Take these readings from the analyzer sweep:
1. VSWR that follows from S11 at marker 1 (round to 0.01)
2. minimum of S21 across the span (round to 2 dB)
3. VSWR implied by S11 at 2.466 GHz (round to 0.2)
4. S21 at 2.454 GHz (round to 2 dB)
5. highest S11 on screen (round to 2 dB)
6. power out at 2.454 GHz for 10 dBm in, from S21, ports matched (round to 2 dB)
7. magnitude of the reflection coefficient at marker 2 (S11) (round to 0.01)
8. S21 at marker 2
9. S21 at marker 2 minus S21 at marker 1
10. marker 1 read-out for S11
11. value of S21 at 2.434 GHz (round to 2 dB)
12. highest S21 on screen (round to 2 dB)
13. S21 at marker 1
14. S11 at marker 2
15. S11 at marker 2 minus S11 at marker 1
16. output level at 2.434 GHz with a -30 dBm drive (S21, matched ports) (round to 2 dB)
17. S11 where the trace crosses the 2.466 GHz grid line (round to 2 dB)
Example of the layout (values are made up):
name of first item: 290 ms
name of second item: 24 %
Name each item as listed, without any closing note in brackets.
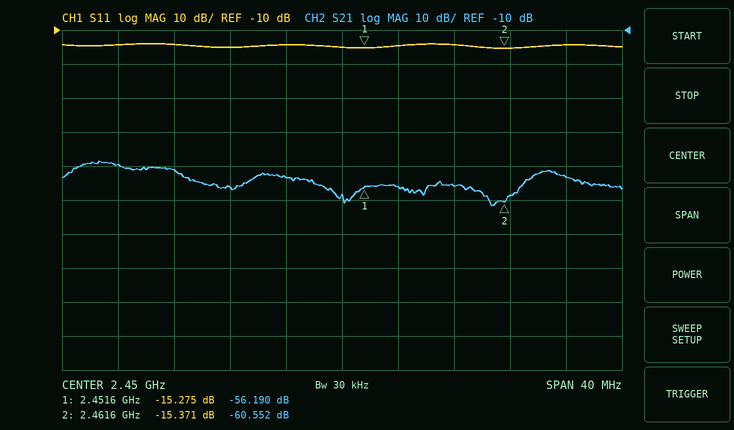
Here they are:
VSWR that follows from S11 at marker 1: 1.42
minimum of S21 across the span: -62 dB
VSWR implied by S11 at 2.466 GHz: 1.4
S21 at 2.454 GHz: -56 dB
highest S11 on screen: -14 dB
power out at 2.454 GHz for 10 dBm in, from S21, ports matched: -46 dBm
magnitude of the reflection coefficient at marker 2 (S11): 0.17
S21 at marker 2: -60.552 dB
S21 at marker 2 minus S21 at marker 1: -4.362 dB
marker 1 read-out for S11: -15.275 dB
value of S21 at 2.434 GHz: -50 dB
highest S21 on screen: -48 dB
S21 at marker 1: -56.190 dB
S11 at marker 2: -15.371 dB
S11 at marker 2 minus S11 at marker 1: -0.096 dB
output level at 2.434 GHz with a -30 dBm drive (S21, matched ports): -80 dBm
S11 where the trace crosses the 2.466 GHz grid line: -14 dB
